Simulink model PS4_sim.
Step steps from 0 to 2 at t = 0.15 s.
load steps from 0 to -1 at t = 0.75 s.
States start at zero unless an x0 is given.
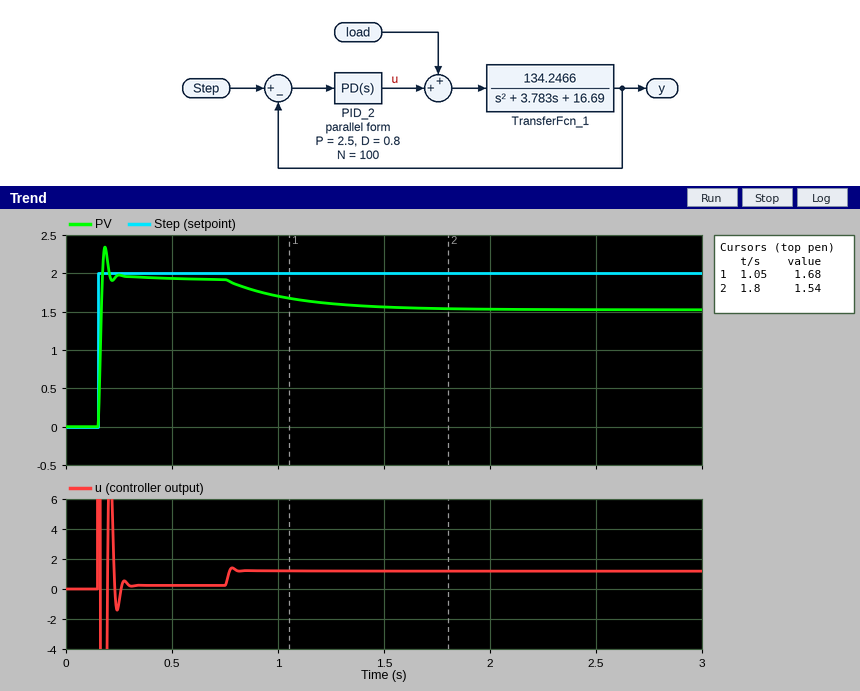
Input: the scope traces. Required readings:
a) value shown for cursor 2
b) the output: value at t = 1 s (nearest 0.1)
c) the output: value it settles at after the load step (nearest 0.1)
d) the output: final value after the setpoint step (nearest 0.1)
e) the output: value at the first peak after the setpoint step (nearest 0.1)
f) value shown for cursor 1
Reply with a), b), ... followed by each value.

a) 1.54
b) 1.7
c) 1.5
d) 1.9
e) 2.3
f) 1.68
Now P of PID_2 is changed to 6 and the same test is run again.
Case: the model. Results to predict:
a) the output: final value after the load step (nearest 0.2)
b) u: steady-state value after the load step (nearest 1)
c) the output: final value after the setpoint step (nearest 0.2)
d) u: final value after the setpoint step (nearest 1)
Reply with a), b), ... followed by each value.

a) 1.8
b) 1
c) 2.0
d) 0
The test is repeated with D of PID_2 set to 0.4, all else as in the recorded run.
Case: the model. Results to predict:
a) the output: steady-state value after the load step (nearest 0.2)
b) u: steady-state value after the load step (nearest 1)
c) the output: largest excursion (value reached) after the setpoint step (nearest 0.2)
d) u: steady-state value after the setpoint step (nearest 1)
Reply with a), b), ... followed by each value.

a) 1.6
b) 1
c) 2.2
d) 0
